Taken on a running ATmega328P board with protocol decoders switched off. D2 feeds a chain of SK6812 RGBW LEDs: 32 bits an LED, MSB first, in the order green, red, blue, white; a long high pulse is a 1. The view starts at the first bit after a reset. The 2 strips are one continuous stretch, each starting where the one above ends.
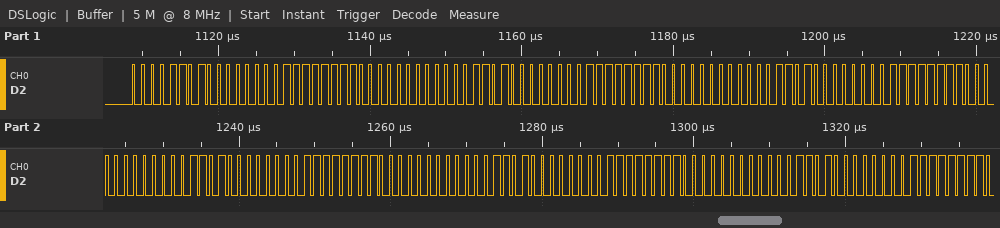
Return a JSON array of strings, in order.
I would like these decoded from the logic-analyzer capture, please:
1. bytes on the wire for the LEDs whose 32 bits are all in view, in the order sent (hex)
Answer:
["0D 00 FF 00 0D 00 FF 00 0D 00 FF 00 0D 00 FF 00 0D 00 FF 00"]
